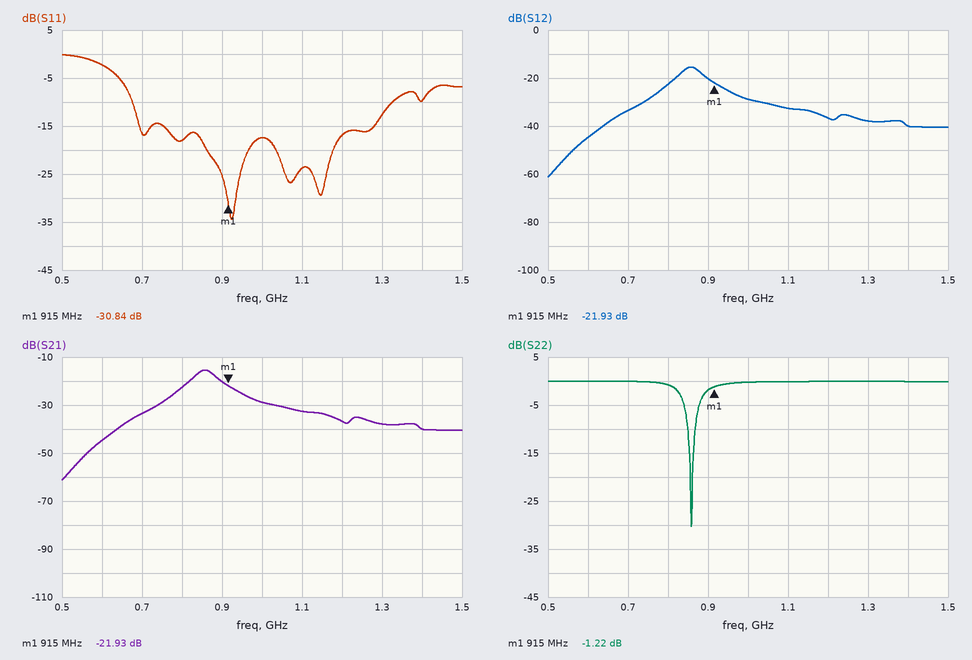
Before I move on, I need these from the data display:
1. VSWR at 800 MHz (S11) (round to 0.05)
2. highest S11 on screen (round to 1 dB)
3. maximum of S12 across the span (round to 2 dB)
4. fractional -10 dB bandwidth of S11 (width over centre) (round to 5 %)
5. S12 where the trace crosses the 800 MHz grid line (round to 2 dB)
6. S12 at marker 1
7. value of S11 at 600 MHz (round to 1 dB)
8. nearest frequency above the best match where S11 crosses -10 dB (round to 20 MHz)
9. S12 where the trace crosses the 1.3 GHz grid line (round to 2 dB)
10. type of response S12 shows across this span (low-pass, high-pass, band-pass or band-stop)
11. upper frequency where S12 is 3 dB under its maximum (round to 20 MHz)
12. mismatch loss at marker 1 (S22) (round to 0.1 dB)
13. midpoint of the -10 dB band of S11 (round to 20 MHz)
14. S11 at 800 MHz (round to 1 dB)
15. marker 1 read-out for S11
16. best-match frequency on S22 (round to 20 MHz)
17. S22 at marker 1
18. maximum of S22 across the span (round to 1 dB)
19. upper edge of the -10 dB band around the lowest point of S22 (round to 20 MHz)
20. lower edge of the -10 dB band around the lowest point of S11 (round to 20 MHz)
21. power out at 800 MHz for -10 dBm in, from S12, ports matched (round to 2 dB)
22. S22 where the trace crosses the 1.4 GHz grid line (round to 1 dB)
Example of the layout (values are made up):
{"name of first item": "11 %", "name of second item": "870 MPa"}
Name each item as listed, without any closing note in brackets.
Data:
{"VSWR at 800 MHz (S11)": "1.30", "highest S11 on screen": "0 dB", "maximum of S12 across the span": "-16 dB", "fractional -10 dB bandwidth of S11 (width over centre)": "65 %", "S12 where the trace crosses the 800 MHz grid line": "-22 dB", "S12 at marker 1": "-21.93 dB", "value of S11 at 600 MHz": "-2 dB", "nearest frequency above the best match where S11 crosses -10 dB": "1.32 GHz", "S12 where the trace crosses the 1.3 GHz grid line": "-38 dB", "type of response S12 shows across this span": "band-pass", "upper frequency where S12 is 3 dB under its maximum": "880 MHz", "mismatch loss at marker 1 (S22)": "6.1 dB", "midpoint of the -10 dB band of S11": "1.00 GHz", "S11 at 800 MHz": "-18 dB", "marker 1 read-out for S11": "-30.84 dB", "best-match frequency on S22": "860 MHz", "S22 at marker 1": "-1.22 dB", "maximum of S22 across the span": "0 dB", "upper edge of the -10 dB band around the lowest point of S22": "860 MHz", "lower edge of the -10 dB band around the lowest point of S11": "680 MHz", "power out at 800 MHz for -10 dBm in, from S12, ports matched": "-32 dBm", "S22 where the trace crosses the 1.4 GHz grid line": "0 dB"}
